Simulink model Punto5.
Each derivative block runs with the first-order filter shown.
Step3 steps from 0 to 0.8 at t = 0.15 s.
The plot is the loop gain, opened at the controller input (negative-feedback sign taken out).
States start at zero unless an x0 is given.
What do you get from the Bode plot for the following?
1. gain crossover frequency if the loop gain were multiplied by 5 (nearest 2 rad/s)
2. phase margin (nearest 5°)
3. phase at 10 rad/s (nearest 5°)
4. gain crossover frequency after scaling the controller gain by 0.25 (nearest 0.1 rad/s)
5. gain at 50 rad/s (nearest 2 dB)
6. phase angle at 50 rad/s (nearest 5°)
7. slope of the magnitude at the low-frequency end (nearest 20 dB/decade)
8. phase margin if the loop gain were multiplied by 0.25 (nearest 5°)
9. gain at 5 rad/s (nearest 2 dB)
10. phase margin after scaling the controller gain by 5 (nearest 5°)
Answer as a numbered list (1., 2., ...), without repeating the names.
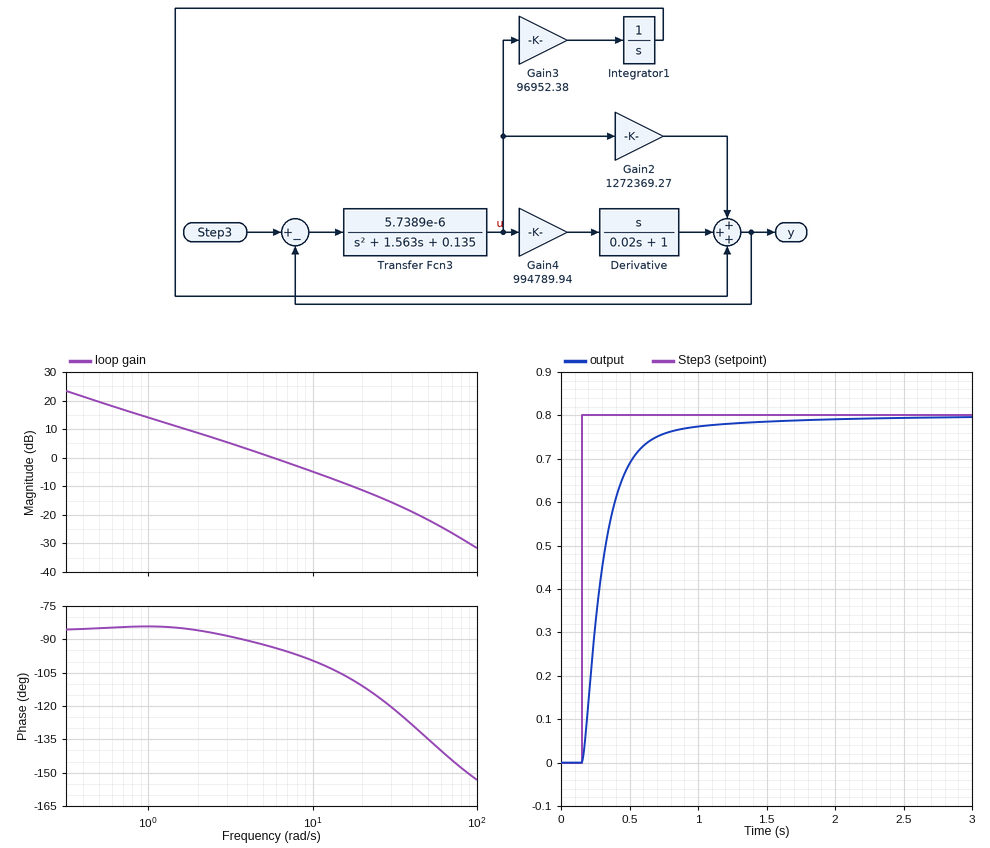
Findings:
1. 26 rad/s
2. 85°
3. -100°
4. 1.3 rad/s
5. -22 dB
6. -135°
7. -20 dB/decade
8. 95°
9. 2 dB
10. 65°
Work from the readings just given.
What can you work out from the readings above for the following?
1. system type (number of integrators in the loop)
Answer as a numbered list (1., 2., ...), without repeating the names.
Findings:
1. 1
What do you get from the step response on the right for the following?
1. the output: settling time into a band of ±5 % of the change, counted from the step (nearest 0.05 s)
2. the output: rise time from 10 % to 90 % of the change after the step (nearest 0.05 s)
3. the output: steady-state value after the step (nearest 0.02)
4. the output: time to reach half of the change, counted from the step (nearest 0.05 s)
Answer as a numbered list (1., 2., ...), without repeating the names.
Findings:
1. 0.60 s
2. 0.40 s
3. 0.80
4. 0.15 s
